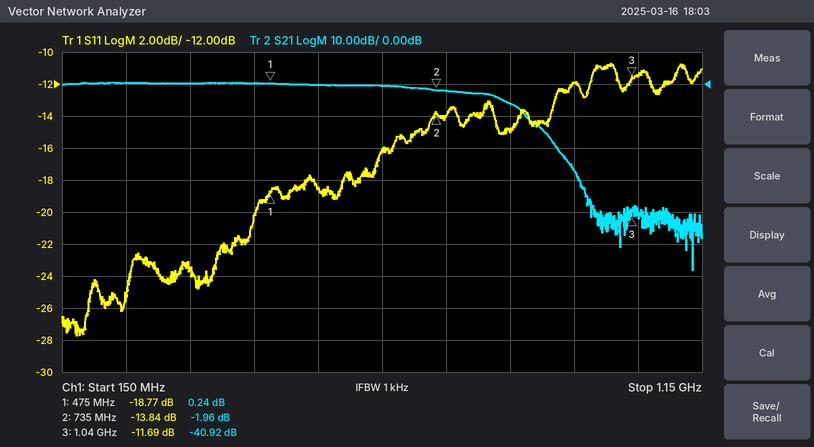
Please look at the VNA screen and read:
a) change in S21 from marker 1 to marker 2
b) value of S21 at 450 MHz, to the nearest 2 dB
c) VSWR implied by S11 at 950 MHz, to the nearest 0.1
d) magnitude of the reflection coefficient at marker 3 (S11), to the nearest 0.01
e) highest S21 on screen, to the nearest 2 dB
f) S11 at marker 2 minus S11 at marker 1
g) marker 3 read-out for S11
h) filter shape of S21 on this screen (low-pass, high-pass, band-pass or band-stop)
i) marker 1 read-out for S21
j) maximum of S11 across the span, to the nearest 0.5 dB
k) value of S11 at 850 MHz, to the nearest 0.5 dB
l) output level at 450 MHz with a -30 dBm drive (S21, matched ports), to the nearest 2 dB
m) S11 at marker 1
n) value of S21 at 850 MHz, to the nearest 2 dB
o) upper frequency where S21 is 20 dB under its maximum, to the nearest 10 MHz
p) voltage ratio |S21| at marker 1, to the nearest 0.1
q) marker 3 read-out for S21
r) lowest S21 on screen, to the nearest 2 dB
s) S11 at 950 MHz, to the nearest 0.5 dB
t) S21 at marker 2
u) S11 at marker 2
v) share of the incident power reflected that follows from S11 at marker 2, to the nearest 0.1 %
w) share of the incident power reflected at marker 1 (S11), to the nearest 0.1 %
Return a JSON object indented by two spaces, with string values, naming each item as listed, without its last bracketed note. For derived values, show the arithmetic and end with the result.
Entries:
{
  "change in S21 from marker 1 to marker 2": "-1.96 − (0.24) = -2.20 dB",
  "value of S21 at 450 MHz, to the nearest 2 dB": "0 dB",
  "VSWR implied by S11 at 950 MHz, to the nearest 0.1": "|Γ| = 10^(-12/20) = 0.2512; VSWR = (1 + 0.2512)/(1 − 0.2512) ≈ 1.7",
  "magnitude of the reflection coefficient at marker 3 (S11), to the nearest 0.01": "10^(-11.69/20) ≈ 0.26",
  "highest S21 on screen, to the nearest 2 dB": "0 dB",
  "S11 at marker 2 minus S11 at marker 1": "-13.84 − (-18.77) = 4.93 dB",
  "marker 3 read-out for S11": "-11.69 dB",
  "filter shape of S21 on this screen": "low-pass",
  "marker 1 read-out for S21": "0.24 dB",
  "maximum of S11 across the span, to the nearest 0.5 dB": "-10.5 dB",
  "value of S11 at 850 MHz, to the nearest 0.5 dB": "-15.0 dB",
  "output level at 450 MHz with a -30 dBm drive (S21, matched ports), to the nearest 2 dB": "-30 dBm + (0 dB) = -30 dBm",
  "S11 at marker 1": "-18.77 dB",
  "value of S21 at 850 MHz, to the nearest 2 dB": "-6 dB",
  "upper frequency where S21 is 20 dB under its maximum, to the nearest 10 MHz": "920 MHz",
  "voltage ratio |S21| at marker 1, to the nearest 0.1": "10^(0.24/20) ≈ 1.0",
  "marker 3 read-out for S21": "-40.92 dB",
  "lowest S21 on screen, to the nearest 2 dB": "-58 dB",
  "S11 at 950 MHz, to the nearest 0.5 dB": "-12.0 dB",
  "S21 at marker 2": "-1.96 dB",
  "S11 at marker 2": "-13.84 dB",
  "share of the incident power reflected that follows from S11 at marker 2, to the nearest 0.1 %": "10^(-13.84/10) ≈ 4.1 %",
  "share of the incident power reflected at marker 1 (S11), to the nearest 0.1 %": "10^(-18.77/10) ≈ 1.3 %"
}
